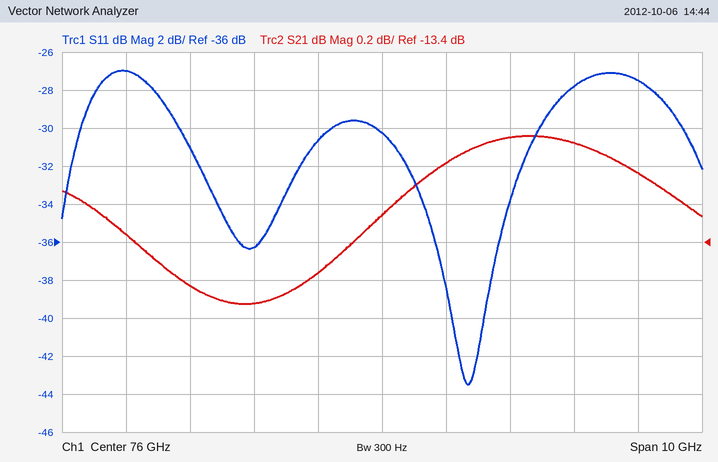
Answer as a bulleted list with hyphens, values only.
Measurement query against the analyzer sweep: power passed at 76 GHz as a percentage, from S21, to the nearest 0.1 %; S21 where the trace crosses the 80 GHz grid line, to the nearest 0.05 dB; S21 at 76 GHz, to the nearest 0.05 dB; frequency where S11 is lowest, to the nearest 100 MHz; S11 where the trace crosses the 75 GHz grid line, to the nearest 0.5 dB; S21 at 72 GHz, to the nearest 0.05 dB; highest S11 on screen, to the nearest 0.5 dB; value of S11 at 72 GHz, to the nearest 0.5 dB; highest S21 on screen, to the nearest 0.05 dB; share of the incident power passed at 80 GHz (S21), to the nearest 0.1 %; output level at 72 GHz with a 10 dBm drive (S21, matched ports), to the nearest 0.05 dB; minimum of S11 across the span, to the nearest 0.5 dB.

- 4.7 %
- -13.05 dB
- -13.25 dB
- 77.3 GHz
- -30.5 dB
- -13.35 dB
- -27.0 dB
- -27.0 dB
- -12.85 dB
- 5.0 %
- -3.35 dBm
- -43.5 dB
